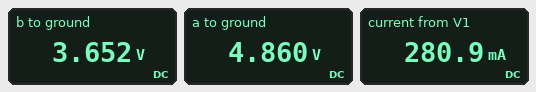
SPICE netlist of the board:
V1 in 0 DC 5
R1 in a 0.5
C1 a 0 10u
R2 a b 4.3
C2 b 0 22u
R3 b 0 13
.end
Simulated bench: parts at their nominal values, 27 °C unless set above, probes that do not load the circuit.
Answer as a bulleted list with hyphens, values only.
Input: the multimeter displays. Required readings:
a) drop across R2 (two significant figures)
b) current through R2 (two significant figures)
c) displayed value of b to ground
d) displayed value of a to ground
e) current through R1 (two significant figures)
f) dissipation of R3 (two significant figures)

- 1.2 V
- 280 mA
- 3.652 V
- 4.860 V
- 280 mA
- 1.0 W
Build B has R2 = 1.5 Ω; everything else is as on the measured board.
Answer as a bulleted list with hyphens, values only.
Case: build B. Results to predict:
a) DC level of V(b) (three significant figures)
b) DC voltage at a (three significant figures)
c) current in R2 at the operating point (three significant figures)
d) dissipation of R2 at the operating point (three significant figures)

- 4.33 V
- 4.83 V
- 333 mA
- 167 mW
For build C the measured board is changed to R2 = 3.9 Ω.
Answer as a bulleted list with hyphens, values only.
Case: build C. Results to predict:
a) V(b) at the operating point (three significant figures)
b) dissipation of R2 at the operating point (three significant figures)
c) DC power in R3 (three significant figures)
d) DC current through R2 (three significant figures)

- 3.74 V
- 322 mW
- 1.07 W
- 287 mA
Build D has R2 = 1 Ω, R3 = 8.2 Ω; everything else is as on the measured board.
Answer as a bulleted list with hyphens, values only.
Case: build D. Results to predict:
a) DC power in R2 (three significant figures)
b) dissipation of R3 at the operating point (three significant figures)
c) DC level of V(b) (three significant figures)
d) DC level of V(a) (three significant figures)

- 266 mW
- 2.18 W
- 4.23 V
- 4.74 V
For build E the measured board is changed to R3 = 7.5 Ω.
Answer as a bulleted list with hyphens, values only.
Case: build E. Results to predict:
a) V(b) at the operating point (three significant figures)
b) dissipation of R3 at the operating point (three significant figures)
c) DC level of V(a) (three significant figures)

- 3.05 V
- 1.24 W
- 4.80 V
